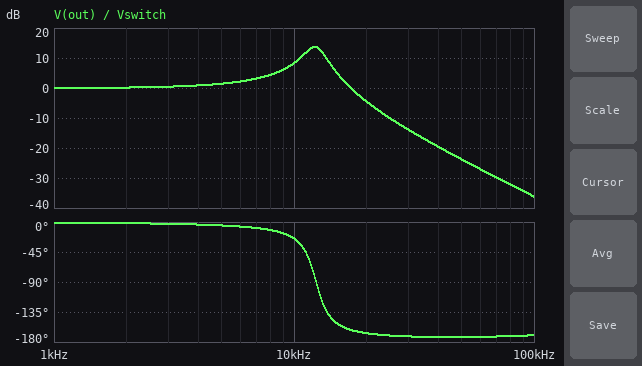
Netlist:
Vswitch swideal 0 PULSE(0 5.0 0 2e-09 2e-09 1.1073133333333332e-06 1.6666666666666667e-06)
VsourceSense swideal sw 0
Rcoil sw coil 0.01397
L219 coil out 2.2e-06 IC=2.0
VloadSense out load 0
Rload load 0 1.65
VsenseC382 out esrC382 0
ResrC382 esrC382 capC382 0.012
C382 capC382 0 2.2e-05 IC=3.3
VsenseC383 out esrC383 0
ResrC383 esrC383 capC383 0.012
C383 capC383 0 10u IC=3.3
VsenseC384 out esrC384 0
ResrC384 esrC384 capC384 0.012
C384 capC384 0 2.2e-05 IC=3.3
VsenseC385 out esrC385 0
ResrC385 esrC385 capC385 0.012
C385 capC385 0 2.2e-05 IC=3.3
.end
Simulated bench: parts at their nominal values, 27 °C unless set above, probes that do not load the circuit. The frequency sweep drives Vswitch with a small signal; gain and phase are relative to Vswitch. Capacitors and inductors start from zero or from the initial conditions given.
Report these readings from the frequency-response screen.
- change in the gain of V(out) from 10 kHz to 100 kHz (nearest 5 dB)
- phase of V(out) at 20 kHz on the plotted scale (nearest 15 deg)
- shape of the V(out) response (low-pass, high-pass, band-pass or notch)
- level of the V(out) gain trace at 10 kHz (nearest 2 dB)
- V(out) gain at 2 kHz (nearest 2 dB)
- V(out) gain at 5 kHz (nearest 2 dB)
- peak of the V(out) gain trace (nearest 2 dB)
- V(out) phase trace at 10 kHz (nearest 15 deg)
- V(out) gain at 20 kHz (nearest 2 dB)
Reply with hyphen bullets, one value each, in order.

- -45 dB
- -165 deg
- low-pass
- 8 dB
- 0 dB
- 2 dB
- 14 dB
- -30 deg
- -4 dB
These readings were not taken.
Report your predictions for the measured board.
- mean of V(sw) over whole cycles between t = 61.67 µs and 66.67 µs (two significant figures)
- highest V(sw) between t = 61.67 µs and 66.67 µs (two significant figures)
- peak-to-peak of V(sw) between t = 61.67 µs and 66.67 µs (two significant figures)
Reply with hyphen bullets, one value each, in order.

- 3.3 V
- 5.0 V
- 5.0 V
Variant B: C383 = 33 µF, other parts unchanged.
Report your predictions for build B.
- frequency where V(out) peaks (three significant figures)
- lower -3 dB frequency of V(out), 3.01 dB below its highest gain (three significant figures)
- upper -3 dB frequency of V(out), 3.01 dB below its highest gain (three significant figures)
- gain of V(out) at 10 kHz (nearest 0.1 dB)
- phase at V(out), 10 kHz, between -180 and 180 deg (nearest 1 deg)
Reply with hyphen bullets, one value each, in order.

- 10.7 kHz
- 9.53 kHz
- 11.8 kHz
- 12.4 dB
- -51 deg
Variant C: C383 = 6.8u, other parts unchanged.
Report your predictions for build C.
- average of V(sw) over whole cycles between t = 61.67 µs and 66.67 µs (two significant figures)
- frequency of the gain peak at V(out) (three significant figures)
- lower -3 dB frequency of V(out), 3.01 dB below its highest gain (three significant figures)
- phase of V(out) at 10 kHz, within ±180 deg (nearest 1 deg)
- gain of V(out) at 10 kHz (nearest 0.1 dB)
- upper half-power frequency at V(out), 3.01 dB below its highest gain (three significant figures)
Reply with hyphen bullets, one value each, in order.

- 3.3 V
- 12.5 kHz
- 11.1 kHz
- -23 deg
- 7.8 dB
- 13.7 kHz
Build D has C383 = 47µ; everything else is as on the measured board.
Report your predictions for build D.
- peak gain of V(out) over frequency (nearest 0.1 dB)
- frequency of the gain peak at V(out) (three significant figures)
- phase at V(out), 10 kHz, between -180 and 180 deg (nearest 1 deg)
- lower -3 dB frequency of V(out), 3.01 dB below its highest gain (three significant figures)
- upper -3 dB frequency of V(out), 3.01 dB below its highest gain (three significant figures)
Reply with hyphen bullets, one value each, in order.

- 13.6 dB
- 10.0 kHz
- -82 deg
- 8.89 kHz
- 11.0 kHz
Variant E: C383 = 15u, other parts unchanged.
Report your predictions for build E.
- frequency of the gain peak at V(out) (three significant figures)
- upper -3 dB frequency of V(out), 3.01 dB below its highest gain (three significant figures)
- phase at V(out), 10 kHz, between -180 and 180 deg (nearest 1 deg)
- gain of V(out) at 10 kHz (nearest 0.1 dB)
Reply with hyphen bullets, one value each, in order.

- 11.8 kHz
- 13.0 kHz
- -28 deg
- 9.2 dB
